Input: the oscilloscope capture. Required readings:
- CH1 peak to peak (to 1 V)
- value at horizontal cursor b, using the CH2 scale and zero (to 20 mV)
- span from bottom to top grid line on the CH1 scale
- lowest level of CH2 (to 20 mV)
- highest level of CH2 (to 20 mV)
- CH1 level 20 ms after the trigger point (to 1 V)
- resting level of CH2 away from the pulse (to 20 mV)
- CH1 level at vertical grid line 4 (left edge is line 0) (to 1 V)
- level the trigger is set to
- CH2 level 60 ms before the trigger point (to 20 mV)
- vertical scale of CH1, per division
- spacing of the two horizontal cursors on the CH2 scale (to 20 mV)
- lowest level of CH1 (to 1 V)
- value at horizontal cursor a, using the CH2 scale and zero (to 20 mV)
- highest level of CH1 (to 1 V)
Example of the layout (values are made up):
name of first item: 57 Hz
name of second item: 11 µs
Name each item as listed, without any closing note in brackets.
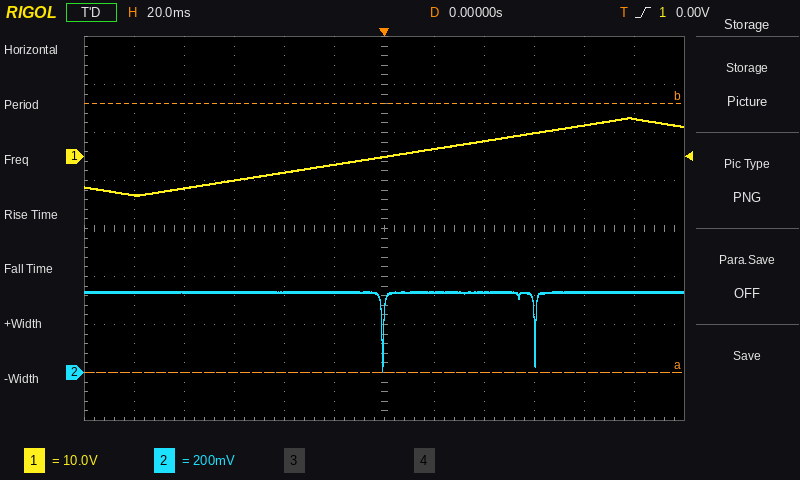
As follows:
CH1 peak to peak: 16 V
value at horizontal cursor b, using the CH2 scale and zero: 1.12 V
span from bottom to top grid line on the CH1 scale: 80 V
lowest level of CH2: 0 mV
highest level of CH2: 340 mV
CH1 level 20 ms after the trigger point: 2 V
resting level of CH2 away from the pulse: 340 mV
CH1 level at vertical grid line 4 (left edge is line 0): -3 V
level the trigger is set to: 0.00 V
CH2 level 60 ms before the trigger point: 340 mV
vertical scale of CH1, per division: 10 V
spacing of the two horizontal cursors on the CH2 scale: 1.12 V
lowest level of CH1: -8 V
value at horizontal cursor a, using the CH2 scale and zero: 0 mV
highest level of CH1: 8 V
